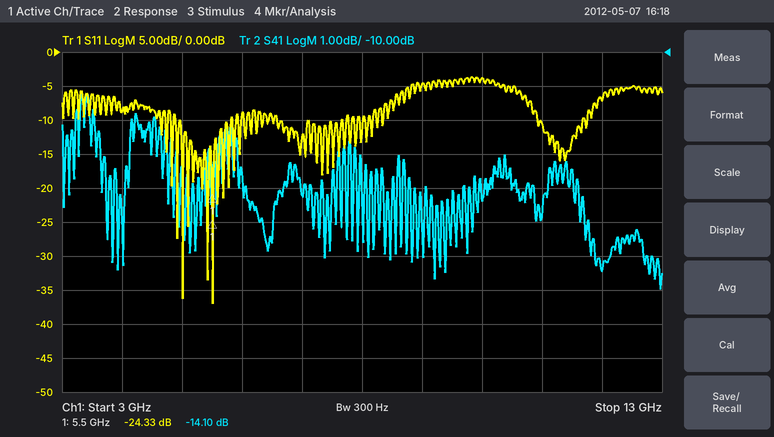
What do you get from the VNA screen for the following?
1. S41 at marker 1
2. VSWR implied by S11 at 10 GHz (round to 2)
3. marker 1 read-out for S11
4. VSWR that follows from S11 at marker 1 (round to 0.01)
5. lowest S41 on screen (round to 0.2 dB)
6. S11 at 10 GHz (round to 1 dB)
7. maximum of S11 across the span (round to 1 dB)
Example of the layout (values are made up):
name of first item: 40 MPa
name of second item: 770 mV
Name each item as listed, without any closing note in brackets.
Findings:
S41 at marker 1: -14.10 dB
VSWR implied by S11 at 10 GHz: 4
marker 1 read-out for S11: -24.33 dB
VSWR that follows from S11 at marker 1: 1.13
lowest S41 on screen: -17.0 dB
S11 at 10 GHz: -4 dB
maximum of S11 across the span: -4 dB
